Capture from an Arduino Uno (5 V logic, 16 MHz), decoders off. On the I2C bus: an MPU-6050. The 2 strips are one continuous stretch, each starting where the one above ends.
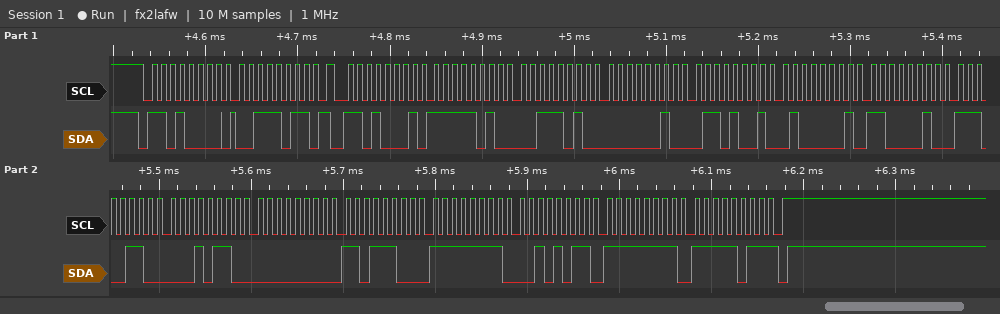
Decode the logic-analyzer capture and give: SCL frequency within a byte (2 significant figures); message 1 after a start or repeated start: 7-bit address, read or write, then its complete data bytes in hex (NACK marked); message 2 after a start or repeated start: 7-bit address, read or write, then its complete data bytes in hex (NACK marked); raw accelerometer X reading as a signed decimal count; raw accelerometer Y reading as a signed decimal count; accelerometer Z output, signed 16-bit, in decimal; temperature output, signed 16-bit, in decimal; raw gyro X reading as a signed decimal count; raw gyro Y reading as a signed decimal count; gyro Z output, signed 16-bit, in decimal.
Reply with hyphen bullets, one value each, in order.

- 100 kHz
- 0x68 write: 3B
- 0x68 read: FA 3A 02 69 41 C2 E6 16 00 DC FF 2B FF FB NACK
- -1478
- 617
- 16834
- -6634
- 220
- -213
- -5
